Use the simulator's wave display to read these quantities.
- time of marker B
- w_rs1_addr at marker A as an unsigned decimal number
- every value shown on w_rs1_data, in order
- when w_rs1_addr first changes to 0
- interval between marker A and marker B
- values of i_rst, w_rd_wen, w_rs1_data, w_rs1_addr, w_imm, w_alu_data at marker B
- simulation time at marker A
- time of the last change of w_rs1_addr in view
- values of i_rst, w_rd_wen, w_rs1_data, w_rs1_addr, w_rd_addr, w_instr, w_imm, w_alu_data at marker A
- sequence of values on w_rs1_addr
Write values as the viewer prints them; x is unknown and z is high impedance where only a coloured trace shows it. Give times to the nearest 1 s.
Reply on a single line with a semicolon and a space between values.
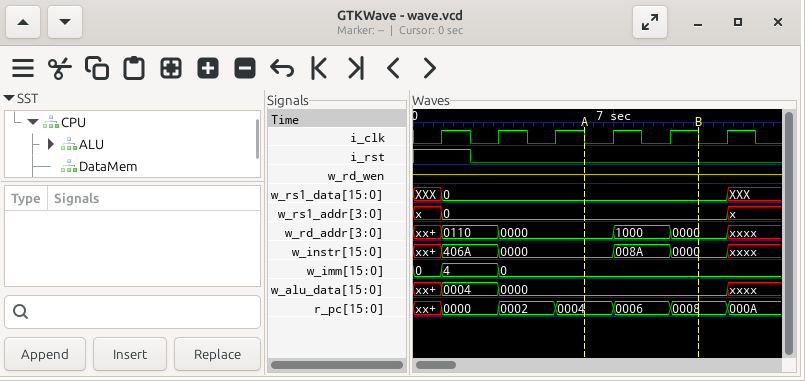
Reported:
10 s; 0; XXX, 0, XXX; 1 s; 4 s; i_rst=0, w_rd_wen=z, w_rs1_data=0, w_rs1_addr=0, w_imm=0, w_alu_data=0000; 6 s; 11 s; i_rst=0, w_rd_wen=z, w_rs1_data=0, w_rs1_addr=0, w_rd_addr=0000, w_instr=0000, w_imm=0, w_alu_data=0000; x, 0, x
